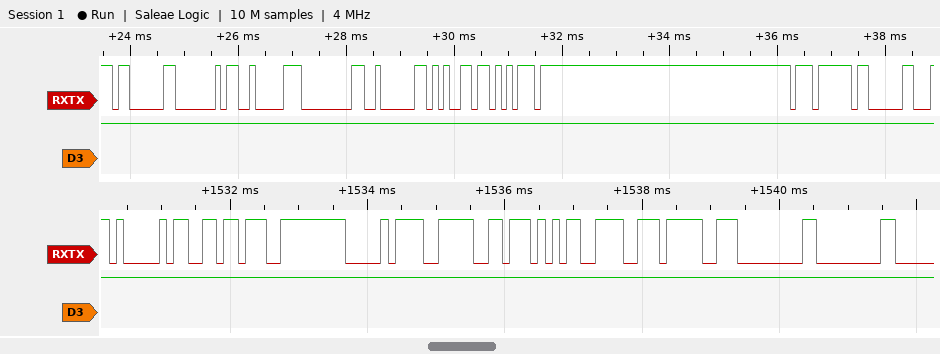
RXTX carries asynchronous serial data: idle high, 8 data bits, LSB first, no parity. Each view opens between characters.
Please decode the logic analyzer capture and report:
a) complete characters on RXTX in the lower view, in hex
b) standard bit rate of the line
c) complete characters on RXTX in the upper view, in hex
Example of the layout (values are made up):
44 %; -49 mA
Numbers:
41, B6, FE, D0, 3E, 57, 9E, 9F, 00, 00; 9600 baud; 03, 40, 82, 00, 02, 65, 75, F7, 03
